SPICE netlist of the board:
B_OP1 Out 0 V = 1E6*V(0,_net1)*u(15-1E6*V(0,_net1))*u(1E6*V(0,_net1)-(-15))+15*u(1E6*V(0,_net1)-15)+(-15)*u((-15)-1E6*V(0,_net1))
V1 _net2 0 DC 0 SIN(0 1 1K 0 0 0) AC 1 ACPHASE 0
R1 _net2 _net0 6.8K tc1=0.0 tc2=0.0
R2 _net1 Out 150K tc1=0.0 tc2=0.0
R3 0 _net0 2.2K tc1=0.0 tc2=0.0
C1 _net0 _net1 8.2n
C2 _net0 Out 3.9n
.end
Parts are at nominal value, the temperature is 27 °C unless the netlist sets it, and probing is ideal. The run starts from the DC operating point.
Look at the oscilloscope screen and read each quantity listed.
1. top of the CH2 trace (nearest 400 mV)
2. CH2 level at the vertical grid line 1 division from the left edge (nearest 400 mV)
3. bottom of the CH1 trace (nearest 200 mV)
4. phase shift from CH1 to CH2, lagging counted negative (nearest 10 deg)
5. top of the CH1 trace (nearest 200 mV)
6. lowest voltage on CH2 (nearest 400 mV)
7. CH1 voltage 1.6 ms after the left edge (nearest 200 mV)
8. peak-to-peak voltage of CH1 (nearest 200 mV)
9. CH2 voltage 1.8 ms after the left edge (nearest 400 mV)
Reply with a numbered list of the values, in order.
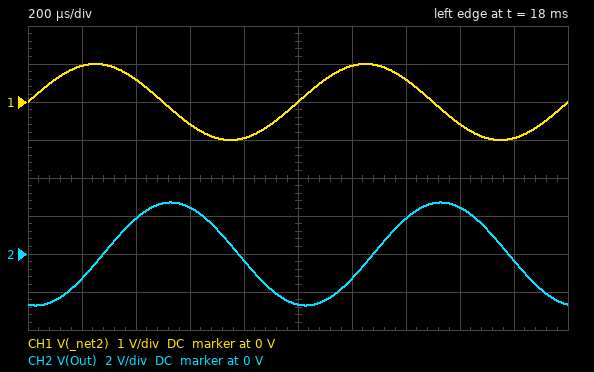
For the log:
1. 2.8 V
2. -1.2 V
3. -1.0 V
4. -100 deg
5. 1.0 V
6. -2.8 V
7. -600 mV
8. 2.0 V
9. -400 mV
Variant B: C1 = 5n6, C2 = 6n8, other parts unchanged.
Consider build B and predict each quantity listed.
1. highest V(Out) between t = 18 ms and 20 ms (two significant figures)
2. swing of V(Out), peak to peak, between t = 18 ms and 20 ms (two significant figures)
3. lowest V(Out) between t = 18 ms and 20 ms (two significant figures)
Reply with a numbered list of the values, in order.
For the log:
1. 2.0 V
2. 4.0 V
3. -2.0 V
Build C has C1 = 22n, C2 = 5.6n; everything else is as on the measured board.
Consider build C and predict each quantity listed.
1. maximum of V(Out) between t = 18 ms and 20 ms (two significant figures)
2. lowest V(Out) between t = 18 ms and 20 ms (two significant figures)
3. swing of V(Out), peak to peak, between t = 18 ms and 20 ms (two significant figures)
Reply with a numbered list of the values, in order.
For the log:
1. 14 V
2. -14 V
3. 28 V
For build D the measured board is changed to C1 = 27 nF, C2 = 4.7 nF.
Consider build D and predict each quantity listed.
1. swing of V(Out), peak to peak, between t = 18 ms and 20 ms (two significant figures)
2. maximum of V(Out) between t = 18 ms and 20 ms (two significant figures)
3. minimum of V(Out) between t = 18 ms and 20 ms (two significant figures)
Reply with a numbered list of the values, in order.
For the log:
1. 30 V
2. 15 V
3. -15 V
